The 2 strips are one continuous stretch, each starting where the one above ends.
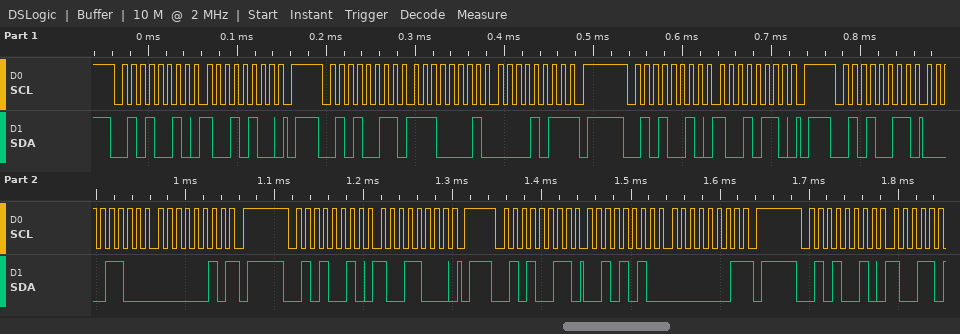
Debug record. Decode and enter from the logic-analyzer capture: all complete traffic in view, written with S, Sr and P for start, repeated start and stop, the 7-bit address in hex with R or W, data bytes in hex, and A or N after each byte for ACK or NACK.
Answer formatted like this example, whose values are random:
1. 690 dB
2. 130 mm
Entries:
1. S 29W A 94 A P S 29R A E1 A 0B N P S 29W A 96 A P S 29R A 0C A 02 N P S 29W A 98 A P S 29R A 2A A 01 N P S 29W A
